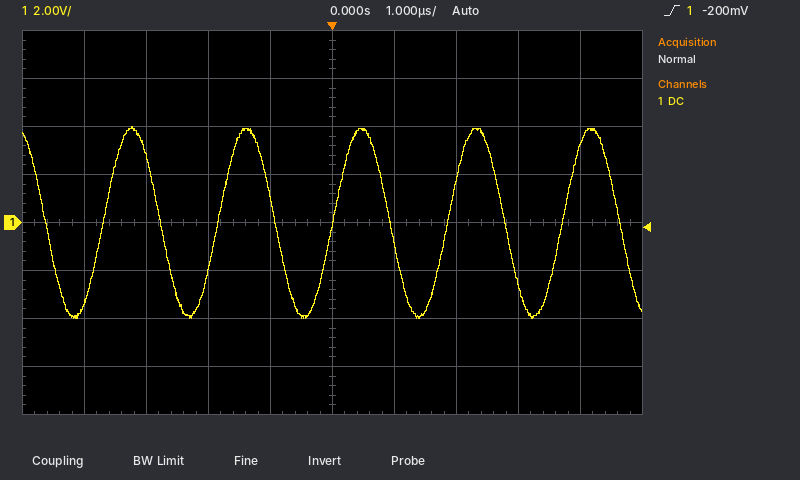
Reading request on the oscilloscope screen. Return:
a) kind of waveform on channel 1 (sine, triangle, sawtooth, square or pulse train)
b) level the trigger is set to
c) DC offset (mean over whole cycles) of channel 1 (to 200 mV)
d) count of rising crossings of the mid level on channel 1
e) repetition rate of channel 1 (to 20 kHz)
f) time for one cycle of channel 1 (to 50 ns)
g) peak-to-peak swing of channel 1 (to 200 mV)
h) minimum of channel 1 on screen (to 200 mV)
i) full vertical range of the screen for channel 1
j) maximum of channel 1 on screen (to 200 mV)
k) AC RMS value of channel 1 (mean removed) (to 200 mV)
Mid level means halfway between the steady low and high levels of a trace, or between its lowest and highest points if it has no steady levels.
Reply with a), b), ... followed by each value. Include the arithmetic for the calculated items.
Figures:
a) sine
b) -200 mV
c) (4.0 V + (-4.0 V)) / 2 ≈ 0.0 V
d) 5
e) 1 / 1.85 µs ≈ 541 kHz, so 540 kHz to the nearest 20 kHz
f) 1.85 µs
g) 4.0 V − (-4.0 V) = 8.0 V
h) -4.0 V
i) 16 V
j) 4.0 V
k) 8.0 V / (2√2) ≈ 2.8 V
